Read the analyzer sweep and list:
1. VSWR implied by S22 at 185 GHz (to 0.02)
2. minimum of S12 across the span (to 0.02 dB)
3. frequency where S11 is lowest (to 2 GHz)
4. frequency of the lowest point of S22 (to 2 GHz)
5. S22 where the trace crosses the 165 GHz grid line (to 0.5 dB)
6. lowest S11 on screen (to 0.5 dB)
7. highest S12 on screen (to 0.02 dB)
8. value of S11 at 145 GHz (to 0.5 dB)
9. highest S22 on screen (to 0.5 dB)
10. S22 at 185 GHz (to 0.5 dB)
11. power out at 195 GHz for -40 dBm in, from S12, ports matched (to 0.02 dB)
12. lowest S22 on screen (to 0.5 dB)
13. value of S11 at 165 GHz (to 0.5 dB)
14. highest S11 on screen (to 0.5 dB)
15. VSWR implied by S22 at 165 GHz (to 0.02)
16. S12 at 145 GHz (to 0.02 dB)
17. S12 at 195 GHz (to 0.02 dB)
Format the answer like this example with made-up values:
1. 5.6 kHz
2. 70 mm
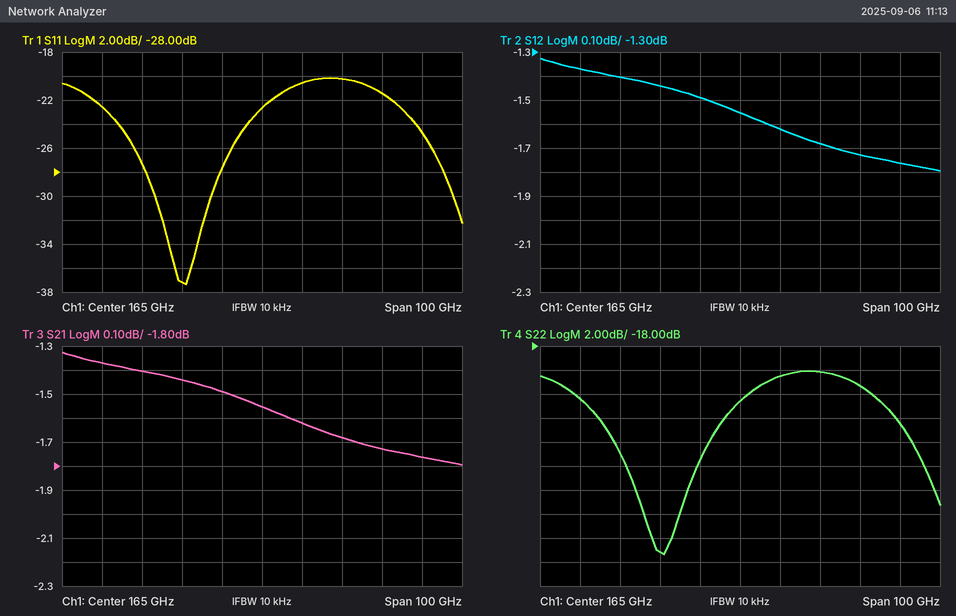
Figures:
1. 1.22
2. -1.80 dB
3. 146 GHz
4. 146 GHz
5. -22.5 dB
6. -37.5 dB
7. -1.32 dB
8. -37.0 dB
9. -20.0 dB
10. -20.0 dB
11. -41.72 dBm
12. -35.5 dB
13. -22.5 dB
14. -20.0 dB
15. 1.16
16. -1.44 dB
17. -1.72 dB
